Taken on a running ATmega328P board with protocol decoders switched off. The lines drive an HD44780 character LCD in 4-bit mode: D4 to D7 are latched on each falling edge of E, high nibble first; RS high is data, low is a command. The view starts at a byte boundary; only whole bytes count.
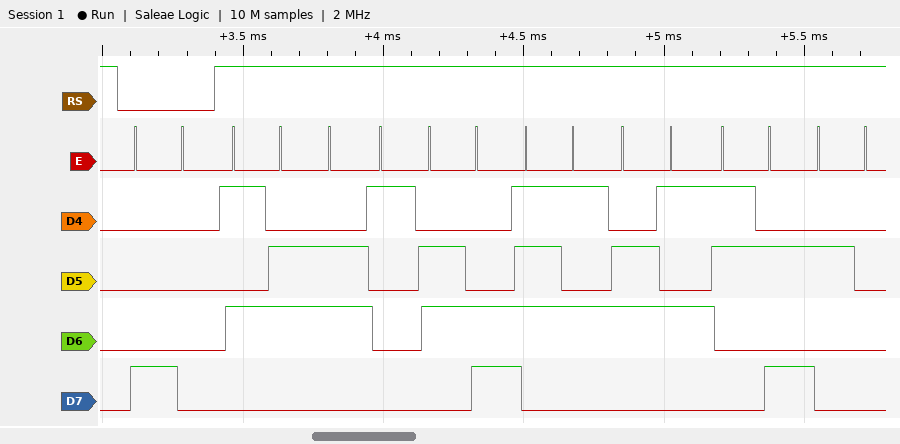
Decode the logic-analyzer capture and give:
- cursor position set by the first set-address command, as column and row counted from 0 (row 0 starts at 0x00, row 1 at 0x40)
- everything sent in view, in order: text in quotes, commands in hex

column 0, row 0
0x80 "Value: "
